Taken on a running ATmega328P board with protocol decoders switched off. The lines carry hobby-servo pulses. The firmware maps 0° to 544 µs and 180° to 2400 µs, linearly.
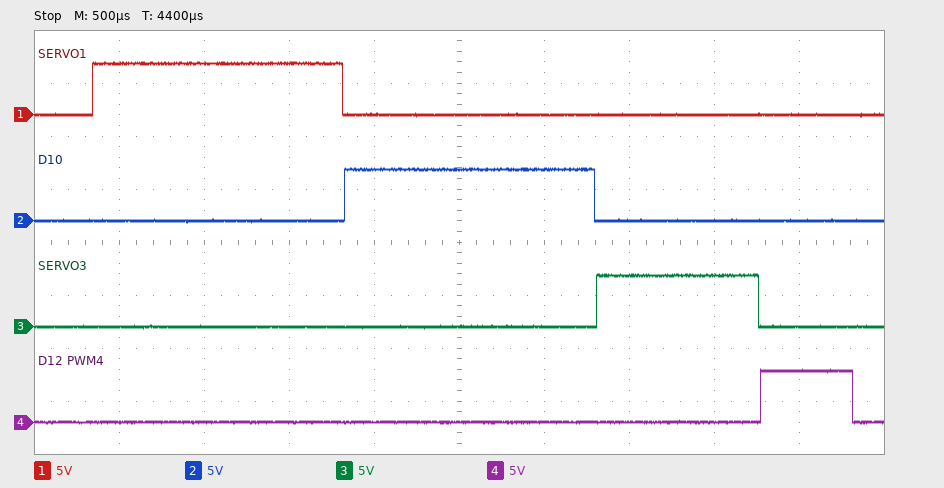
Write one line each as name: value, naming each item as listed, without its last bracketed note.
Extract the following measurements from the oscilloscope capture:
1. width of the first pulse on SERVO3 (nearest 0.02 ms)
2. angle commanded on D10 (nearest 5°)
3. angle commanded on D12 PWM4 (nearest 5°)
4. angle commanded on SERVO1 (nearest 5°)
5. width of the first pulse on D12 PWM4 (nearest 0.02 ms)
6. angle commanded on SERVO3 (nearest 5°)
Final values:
width of the first pulse on SERVO3: 0.96 ms
angle commanded on D10: 90°
angle commanded on D12 PWM4: 0°
angle commanded on SERVO1: 90°
width of the first pulse on D12 PWM4: 0.54 ms
angle commanded on SERVO3: 40°
